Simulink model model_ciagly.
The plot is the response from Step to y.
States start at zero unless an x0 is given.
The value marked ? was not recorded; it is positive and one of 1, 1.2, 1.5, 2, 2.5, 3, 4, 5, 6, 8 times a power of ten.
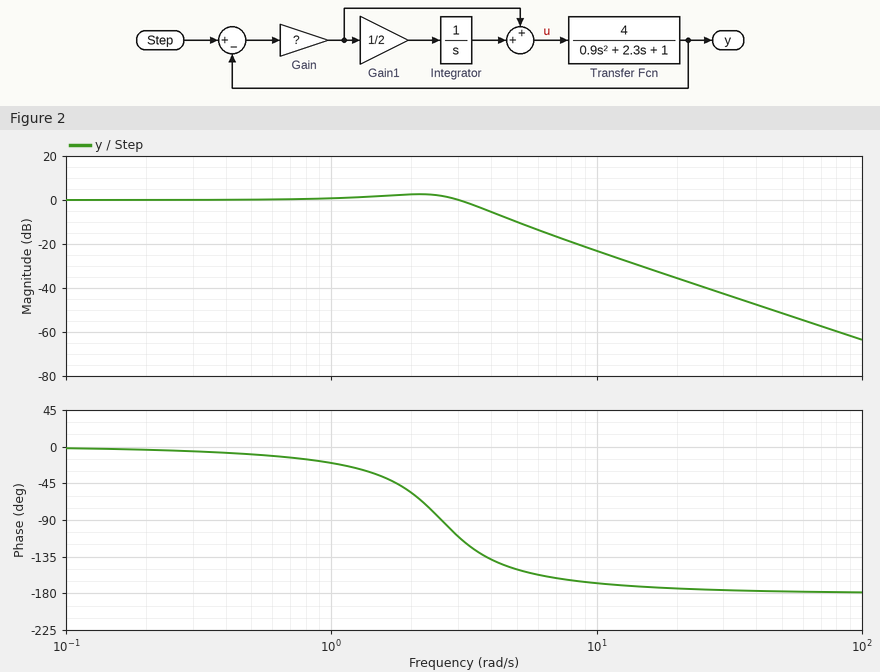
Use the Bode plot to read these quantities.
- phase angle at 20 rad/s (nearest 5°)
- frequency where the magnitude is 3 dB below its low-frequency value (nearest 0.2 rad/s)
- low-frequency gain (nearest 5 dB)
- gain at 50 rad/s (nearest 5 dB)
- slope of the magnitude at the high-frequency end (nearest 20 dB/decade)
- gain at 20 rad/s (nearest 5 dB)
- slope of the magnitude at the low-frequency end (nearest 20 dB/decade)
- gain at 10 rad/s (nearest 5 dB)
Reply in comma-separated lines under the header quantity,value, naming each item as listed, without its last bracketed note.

quantity,value
phase angle at 20 rad/s,-175°
frequency where the magnitude is 3 dB below its low-frequency value,3.6 rad/s
low-frequency gain,0 dB
gain at 50 rad/s,-50 dB
slope of the magnitude at the high-frequency end,-40 dB/decade
gain at 20 rad/s,-35 dB
slope of the magnitude at the low-frequency end,0 dB/decade
gain at 10 rad/s,-25 dB
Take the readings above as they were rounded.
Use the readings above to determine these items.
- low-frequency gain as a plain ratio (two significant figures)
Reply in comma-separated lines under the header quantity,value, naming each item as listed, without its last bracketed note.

quantity,value
low-frequency gain as a plain ratio,1.0
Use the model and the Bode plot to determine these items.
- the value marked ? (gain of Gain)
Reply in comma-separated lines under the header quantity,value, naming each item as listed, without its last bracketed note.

quantity,value
the value marked ?,1.5
